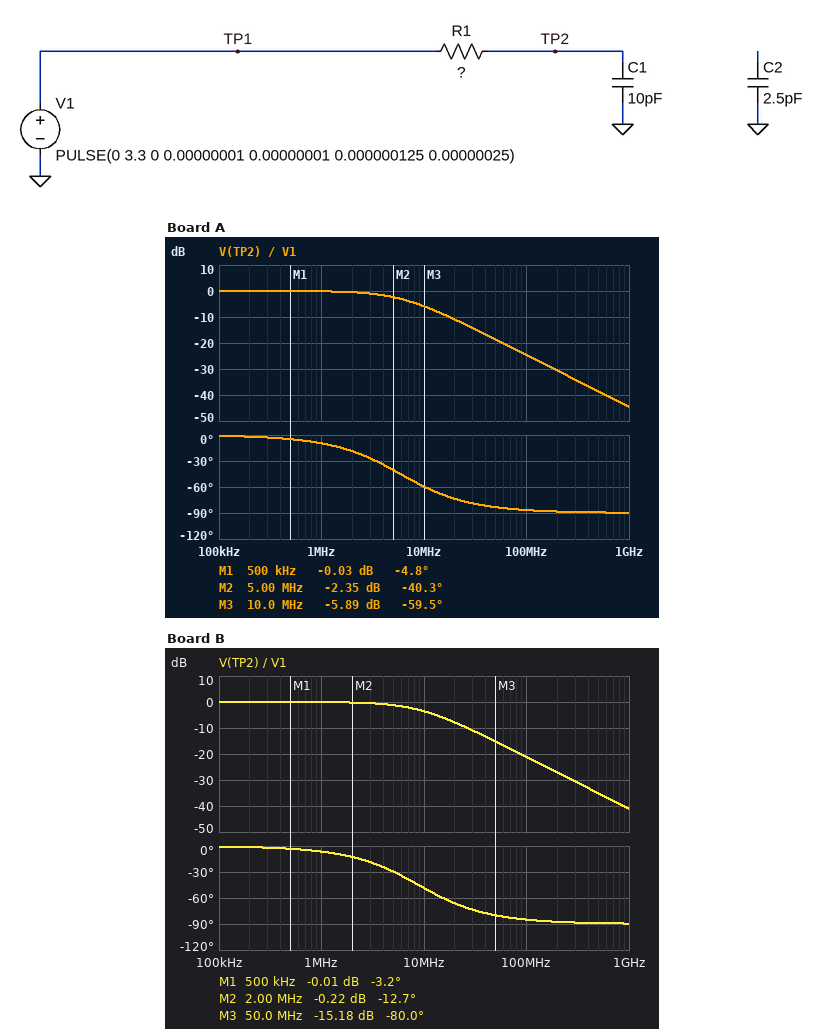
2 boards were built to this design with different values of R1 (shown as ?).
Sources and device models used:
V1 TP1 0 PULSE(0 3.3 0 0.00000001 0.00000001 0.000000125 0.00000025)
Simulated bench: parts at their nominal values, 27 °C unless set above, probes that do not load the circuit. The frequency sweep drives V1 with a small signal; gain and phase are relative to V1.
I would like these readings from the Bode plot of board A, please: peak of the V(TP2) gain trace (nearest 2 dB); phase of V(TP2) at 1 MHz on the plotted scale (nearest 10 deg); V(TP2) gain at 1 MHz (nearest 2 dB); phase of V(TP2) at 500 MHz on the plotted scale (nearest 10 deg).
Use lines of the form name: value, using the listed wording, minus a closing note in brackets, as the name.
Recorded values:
peak of the V(TP2) gain trace: 0 dB
phase of V(TP2) at 1 MHz on the plotted scale: -10 deg
V(TP2) gain at 1 MHz: 0 dB
phase of V(TP2) at 500 MHz on the plotted scale: -90 deg
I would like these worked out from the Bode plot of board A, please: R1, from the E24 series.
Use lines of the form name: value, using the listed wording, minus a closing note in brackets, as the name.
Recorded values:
R1, from the E24 series: 2.7 kΩ
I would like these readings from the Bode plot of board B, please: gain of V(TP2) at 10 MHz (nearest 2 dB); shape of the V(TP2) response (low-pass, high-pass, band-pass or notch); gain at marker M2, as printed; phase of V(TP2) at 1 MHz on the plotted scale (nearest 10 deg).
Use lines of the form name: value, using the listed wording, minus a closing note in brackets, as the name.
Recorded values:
gain of V(TP2) at 10 MHz: -4 dB
shape of the V(TP2) response: low-pass
gain at marker M2, as printed: -0.22 dB
phase of V(TP2) at 1 MHz on the plotted scale: -10 deg
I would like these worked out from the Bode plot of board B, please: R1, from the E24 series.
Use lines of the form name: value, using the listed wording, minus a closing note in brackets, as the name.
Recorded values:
R1, from the E24 series: 1.8 kΩ
